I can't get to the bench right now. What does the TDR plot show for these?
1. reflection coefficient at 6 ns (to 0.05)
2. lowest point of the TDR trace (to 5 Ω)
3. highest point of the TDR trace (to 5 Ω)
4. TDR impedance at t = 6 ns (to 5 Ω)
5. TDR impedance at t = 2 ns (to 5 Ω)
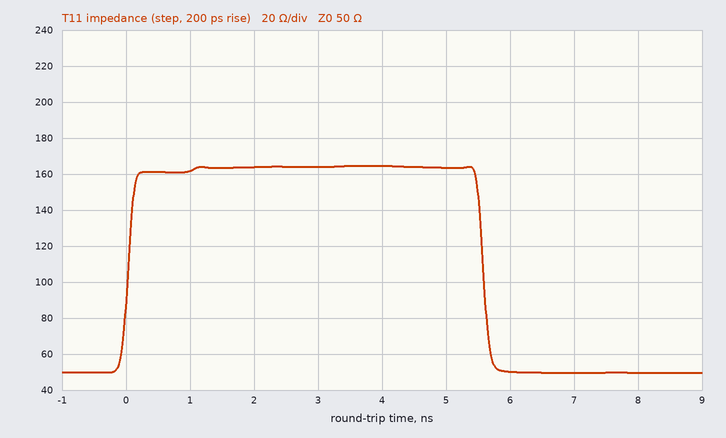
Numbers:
0.00
50 Ω
165 Ω
50 Ω
165 Ω
